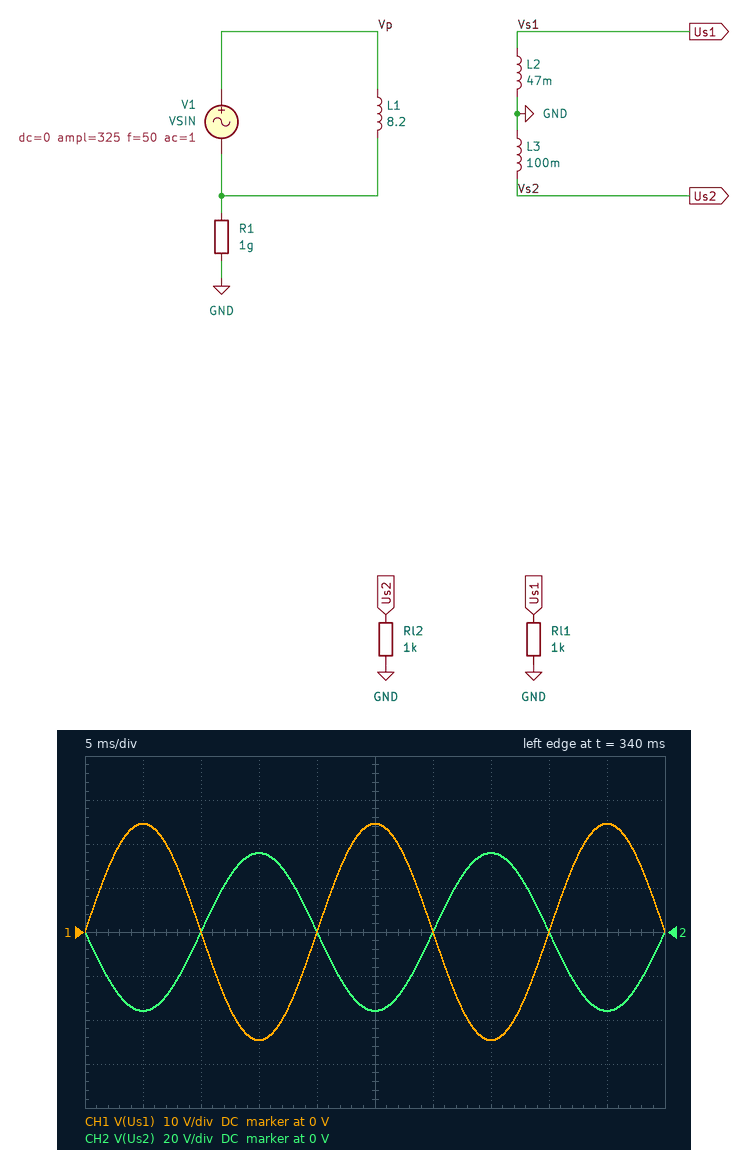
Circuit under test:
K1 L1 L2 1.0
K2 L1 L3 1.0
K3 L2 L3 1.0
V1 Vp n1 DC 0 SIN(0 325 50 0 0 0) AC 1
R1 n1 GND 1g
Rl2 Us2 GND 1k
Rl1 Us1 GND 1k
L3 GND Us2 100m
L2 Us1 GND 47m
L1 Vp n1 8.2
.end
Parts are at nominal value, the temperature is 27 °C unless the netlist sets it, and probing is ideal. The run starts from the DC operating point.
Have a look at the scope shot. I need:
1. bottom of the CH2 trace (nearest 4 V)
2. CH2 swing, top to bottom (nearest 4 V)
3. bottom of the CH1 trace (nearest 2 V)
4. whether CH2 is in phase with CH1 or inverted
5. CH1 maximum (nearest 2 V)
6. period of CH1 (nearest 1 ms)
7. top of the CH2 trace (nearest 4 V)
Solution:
-36 V
72 V
-24 V
inverted
24 V
20 ms
36 V
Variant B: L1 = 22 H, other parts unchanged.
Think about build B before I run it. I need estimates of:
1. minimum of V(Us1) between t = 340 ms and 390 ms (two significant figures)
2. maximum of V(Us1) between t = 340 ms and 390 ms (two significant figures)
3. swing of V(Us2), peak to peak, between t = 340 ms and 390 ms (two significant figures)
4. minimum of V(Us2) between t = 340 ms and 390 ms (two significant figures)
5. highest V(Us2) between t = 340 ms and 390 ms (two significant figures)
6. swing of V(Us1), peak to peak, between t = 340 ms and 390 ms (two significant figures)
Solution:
-15 V
15 V
44 V
-22 V
22 V
30 V
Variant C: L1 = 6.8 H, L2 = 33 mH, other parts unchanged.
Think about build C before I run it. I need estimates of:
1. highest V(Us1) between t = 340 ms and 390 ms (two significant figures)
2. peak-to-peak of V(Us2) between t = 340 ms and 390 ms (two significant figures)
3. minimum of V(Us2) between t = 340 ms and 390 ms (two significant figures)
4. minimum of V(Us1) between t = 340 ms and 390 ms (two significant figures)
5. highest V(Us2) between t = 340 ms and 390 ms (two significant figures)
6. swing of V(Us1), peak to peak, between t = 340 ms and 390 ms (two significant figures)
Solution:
23 V
79 V
-39 V
-23 V
39 V
45 V
